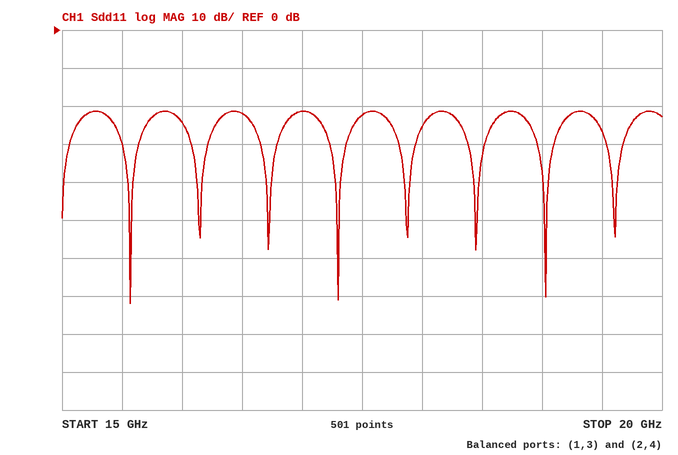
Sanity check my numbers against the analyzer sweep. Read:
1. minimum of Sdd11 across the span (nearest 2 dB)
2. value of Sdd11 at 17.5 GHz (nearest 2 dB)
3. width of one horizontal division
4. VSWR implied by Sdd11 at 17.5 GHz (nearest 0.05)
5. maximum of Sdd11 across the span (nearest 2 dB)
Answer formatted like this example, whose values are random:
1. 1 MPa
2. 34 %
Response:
1. -72 dB
2. -22 dB
3. 500 MHz
4. 1.15
5. -22 dB
